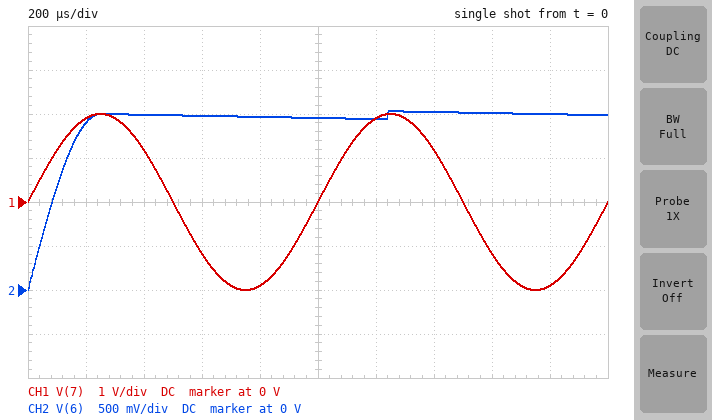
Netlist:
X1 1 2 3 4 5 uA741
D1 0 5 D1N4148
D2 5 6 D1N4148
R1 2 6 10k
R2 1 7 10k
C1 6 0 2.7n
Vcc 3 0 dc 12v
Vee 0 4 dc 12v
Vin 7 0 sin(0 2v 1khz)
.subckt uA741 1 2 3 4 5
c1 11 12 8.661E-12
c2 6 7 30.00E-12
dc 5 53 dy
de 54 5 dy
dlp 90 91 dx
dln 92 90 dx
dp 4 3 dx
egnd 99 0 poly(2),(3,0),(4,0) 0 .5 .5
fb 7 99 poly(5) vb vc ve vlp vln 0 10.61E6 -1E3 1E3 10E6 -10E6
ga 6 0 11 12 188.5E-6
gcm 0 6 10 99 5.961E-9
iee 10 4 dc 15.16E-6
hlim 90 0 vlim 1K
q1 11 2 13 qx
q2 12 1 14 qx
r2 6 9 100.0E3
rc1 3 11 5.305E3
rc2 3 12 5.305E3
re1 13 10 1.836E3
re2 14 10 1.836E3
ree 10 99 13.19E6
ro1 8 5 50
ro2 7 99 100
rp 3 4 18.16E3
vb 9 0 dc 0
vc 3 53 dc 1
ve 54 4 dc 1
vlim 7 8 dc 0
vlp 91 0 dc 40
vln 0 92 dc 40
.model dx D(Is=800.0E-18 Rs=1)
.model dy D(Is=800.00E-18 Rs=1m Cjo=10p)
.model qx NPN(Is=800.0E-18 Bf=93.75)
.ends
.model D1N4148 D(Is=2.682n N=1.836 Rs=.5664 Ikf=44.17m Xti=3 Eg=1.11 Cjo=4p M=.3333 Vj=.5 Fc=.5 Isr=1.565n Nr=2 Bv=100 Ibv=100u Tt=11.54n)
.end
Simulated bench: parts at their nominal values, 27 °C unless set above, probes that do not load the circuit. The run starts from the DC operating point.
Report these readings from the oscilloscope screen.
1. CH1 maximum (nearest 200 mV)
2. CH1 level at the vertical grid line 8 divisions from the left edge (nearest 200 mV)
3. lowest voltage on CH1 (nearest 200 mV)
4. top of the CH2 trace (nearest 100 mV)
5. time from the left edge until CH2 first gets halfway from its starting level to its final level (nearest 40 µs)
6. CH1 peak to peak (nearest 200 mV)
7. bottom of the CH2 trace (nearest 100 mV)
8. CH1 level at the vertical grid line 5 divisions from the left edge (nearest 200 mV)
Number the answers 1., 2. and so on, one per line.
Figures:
1. 2.0 V
2. -1.2 V
3. -2.0 V
4. 2.0 V
5. 80 µs
6. 4.0 V
7. 0 V
8. 0 V
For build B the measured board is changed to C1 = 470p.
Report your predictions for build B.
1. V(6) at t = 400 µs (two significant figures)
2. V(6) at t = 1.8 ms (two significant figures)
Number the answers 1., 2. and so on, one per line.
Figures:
1. 1.9 V
2. 1.8 V
